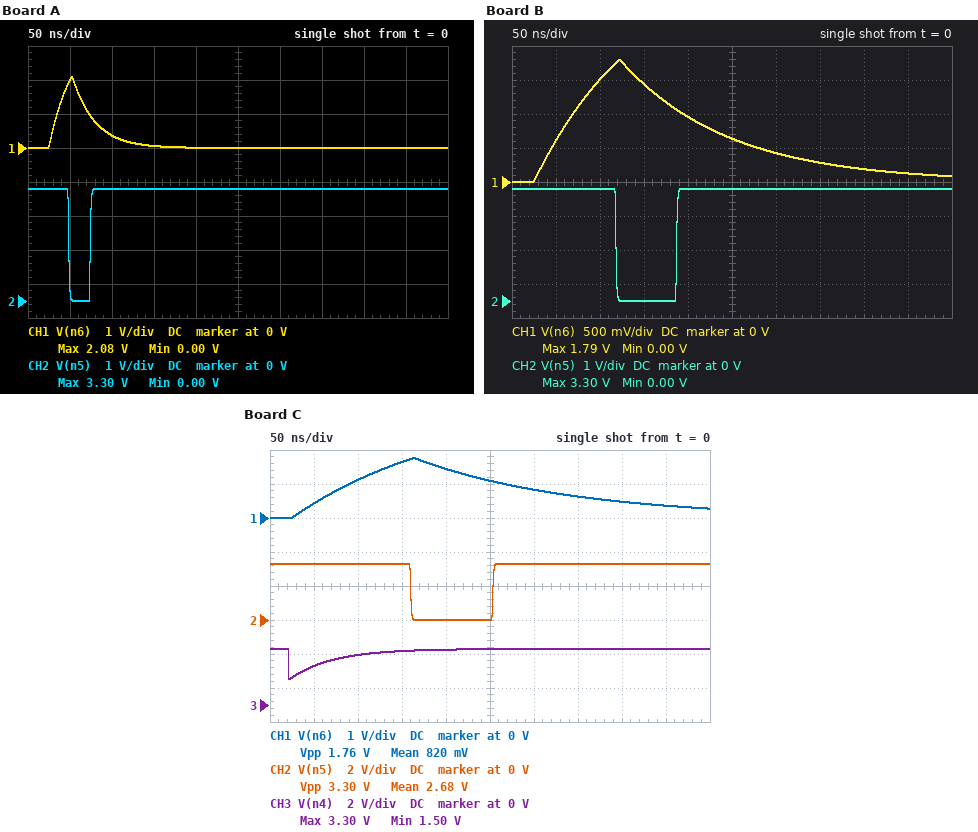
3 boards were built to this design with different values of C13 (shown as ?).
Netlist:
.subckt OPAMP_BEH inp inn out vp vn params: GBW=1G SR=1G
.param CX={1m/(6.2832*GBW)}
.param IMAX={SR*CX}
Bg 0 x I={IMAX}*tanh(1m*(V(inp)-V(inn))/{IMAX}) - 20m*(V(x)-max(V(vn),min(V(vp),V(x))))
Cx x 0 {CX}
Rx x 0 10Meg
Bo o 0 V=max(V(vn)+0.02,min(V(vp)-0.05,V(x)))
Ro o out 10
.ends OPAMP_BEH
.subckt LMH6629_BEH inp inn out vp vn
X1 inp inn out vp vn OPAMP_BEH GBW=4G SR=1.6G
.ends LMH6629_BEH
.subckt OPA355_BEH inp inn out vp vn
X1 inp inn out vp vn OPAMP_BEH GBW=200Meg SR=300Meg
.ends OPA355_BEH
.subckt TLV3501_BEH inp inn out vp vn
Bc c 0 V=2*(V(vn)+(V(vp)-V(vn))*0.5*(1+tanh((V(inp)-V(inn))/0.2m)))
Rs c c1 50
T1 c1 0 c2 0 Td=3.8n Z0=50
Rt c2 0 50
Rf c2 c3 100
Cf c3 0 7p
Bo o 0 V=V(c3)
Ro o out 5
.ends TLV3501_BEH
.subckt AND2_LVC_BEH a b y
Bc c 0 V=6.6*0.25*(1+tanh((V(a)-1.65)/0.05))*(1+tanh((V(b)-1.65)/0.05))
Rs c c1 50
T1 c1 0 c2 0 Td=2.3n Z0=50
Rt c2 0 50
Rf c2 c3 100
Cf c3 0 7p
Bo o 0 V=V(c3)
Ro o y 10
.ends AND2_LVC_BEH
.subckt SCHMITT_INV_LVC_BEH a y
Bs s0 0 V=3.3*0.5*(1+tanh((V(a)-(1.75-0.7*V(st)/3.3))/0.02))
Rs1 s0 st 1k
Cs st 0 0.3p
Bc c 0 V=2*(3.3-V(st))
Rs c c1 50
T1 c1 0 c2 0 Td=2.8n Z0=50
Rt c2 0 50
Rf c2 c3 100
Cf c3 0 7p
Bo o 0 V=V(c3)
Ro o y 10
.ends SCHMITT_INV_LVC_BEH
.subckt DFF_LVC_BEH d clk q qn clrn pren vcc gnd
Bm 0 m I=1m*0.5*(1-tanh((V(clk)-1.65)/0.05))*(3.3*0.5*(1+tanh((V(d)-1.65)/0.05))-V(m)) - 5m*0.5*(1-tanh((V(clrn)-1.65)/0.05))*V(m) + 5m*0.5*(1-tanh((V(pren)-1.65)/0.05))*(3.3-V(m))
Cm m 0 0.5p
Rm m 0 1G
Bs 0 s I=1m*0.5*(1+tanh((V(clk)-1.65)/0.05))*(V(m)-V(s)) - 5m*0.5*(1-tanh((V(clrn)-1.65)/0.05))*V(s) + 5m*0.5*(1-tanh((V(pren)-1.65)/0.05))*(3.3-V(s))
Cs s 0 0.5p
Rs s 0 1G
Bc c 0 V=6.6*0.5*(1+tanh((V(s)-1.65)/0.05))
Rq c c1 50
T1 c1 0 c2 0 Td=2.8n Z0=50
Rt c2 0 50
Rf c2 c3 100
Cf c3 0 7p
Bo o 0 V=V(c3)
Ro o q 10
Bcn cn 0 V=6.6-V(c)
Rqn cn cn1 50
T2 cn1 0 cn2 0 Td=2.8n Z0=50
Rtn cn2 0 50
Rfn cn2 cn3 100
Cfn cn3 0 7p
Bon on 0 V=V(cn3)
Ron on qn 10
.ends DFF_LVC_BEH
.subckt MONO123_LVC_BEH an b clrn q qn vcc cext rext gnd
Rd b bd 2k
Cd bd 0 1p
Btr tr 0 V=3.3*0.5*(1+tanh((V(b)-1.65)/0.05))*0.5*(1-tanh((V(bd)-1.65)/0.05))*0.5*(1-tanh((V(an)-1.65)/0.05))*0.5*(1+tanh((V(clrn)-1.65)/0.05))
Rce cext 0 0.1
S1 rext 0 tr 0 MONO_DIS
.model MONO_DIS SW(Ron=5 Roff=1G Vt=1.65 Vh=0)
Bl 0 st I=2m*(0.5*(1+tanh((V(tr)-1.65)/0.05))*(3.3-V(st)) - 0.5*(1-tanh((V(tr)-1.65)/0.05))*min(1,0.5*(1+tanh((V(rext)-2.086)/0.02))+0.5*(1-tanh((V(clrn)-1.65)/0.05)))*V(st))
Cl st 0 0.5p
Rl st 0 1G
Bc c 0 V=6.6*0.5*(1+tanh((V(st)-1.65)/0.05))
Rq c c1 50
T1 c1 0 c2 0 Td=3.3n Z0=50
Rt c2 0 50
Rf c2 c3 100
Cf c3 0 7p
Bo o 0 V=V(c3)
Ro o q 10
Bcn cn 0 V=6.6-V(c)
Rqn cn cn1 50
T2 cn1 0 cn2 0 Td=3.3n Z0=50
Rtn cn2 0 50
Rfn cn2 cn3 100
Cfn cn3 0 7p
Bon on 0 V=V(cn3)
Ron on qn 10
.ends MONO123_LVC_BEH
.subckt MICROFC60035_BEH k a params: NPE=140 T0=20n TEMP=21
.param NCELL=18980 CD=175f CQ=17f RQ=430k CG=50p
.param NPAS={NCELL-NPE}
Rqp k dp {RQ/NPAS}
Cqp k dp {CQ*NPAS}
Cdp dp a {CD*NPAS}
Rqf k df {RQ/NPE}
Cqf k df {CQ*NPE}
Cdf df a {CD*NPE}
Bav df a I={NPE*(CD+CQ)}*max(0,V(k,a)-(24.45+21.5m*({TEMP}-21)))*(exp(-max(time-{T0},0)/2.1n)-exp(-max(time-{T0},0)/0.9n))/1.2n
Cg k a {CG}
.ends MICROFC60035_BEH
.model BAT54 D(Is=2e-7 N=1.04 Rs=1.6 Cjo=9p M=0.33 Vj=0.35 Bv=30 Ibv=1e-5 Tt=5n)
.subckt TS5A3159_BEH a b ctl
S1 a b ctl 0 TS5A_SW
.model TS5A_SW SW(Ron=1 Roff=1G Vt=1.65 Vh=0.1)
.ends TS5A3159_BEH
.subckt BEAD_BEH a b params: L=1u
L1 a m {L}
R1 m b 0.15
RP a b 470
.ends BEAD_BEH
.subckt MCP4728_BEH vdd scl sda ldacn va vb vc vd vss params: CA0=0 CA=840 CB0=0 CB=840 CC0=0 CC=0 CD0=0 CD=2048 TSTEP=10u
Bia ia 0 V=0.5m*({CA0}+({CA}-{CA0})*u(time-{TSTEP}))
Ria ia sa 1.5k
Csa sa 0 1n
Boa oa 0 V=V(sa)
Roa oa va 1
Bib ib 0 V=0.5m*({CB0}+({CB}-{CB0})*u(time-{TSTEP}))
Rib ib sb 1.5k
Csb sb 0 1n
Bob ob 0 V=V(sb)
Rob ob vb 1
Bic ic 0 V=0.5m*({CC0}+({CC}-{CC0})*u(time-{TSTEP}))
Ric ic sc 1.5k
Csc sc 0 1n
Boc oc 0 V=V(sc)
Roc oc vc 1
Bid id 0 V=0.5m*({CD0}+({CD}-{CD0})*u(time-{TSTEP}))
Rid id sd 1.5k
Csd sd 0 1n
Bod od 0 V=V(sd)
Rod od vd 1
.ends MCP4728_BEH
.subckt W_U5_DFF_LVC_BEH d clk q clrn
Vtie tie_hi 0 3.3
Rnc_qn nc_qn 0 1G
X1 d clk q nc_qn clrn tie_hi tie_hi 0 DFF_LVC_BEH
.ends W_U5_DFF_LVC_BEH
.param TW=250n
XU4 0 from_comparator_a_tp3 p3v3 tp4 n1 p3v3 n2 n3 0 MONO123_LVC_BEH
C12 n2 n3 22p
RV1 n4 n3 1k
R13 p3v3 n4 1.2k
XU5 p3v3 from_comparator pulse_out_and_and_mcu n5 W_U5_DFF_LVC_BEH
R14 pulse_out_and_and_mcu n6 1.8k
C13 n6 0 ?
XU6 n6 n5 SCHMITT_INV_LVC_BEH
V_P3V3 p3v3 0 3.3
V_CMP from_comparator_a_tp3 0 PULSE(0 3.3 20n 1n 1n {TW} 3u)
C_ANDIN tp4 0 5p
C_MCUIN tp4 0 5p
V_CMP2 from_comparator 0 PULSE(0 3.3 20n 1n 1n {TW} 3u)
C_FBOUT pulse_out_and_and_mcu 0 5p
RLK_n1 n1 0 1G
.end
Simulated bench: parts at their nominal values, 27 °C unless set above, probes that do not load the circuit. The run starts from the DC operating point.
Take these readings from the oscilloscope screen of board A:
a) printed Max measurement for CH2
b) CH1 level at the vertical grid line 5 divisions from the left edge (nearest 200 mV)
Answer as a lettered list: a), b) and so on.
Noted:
a) 3.30 V
b) 0 V
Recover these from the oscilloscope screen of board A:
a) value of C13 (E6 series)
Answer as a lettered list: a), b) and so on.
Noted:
a) 15 pF
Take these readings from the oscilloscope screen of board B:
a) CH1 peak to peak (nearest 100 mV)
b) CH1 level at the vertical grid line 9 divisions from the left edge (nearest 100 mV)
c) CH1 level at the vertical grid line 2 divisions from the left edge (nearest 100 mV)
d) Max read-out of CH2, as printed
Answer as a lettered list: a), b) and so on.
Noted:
a) 1.8 V
b) 100 mV
c) 1.5 V
d) 3.30 V
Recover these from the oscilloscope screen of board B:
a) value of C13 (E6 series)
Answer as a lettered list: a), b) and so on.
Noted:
a) 68 pF
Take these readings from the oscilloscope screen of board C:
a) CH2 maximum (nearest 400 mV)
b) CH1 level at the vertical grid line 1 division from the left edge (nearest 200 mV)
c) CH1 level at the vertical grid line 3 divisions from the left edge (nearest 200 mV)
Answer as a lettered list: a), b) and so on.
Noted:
a) 3.2 V
b) 400 mV
c) 1.6 V
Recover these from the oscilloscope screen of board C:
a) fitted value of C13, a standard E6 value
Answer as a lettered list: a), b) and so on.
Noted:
a) 100 pF
